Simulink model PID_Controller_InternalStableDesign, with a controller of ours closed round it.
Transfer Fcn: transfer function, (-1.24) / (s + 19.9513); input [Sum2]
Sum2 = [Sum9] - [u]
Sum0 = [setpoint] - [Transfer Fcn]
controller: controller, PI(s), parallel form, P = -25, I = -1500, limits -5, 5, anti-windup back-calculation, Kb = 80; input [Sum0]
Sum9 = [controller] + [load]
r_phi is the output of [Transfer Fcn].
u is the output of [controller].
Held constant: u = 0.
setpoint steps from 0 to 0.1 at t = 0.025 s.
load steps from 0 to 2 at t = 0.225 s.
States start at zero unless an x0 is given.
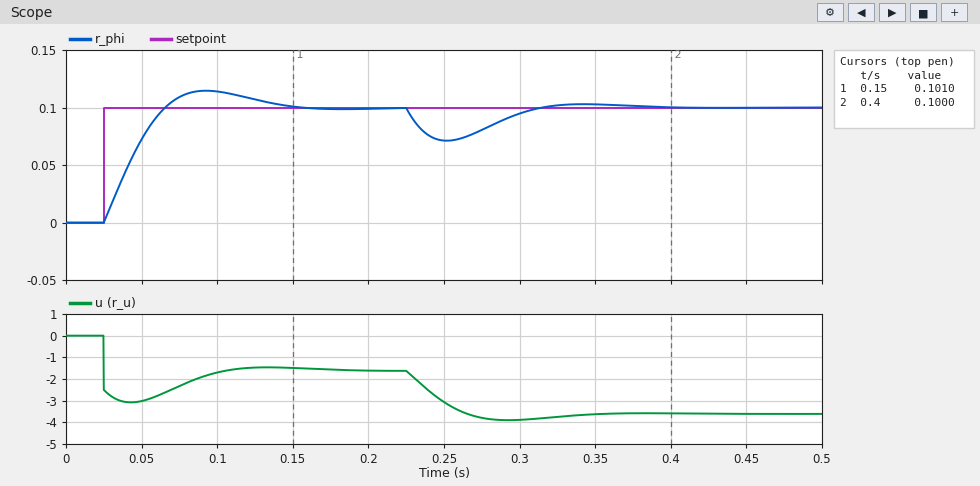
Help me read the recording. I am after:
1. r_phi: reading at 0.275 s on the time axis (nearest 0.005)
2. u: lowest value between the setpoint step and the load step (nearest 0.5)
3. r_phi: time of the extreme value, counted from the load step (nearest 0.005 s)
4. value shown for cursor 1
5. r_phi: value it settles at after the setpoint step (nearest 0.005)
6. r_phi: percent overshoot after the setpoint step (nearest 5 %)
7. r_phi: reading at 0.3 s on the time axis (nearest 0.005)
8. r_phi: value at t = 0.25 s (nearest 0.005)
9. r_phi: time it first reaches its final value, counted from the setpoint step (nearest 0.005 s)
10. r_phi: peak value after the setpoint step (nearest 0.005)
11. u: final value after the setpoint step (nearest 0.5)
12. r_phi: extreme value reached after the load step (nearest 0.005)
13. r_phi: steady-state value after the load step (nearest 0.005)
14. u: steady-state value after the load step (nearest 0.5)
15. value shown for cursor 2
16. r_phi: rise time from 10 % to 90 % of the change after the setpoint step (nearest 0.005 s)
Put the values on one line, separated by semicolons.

0.080; -3.0; 0.025 s; 0.1010; 0.100; 15 %; 0.095; 0.070; 0.040 s; 0.115; -1.5; 0.070; 0.100; -3.5; 0.1000; 0.030 s
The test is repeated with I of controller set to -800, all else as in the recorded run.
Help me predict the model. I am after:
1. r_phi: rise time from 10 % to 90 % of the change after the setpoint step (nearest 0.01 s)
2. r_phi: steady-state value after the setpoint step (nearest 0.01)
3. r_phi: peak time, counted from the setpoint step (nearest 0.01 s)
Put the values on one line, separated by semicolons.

0.05 s; 0.10; 0.10 s
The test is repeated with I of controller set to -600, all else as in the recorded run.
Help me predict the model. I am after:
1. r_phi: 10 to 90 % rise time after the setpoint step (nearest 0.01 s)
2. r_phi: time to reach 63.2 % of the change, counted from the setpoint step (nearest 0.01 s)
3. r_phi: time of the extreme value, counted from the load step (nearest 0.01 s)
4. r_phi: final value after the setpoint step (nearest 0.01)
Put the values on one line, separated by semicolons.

0.06 s; 0.03 s; 0.04 s; 0.10
